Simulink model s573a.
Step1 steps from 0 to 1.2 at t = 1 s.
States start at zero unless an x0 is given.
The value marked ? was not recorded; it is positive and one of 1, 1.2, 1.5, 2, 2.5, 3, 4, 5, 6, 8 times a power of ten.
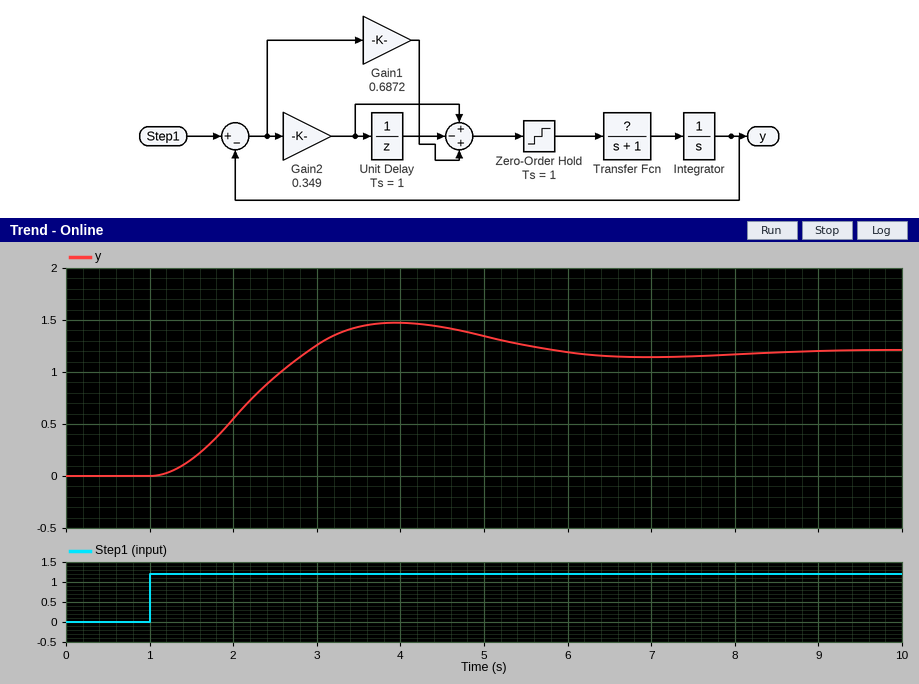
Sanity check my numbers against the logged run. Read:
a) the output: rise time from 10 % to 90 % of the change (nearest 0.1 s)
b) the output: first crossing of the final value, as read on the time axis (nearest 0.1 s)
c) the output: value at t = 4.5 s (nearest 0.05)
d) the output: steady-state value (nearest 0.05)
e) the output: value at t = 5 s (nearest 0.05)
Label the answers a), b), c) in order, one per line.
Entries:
a) 1.3 s
b) 2.9 s
c) 1.45
d) 1.20
e) 1.35
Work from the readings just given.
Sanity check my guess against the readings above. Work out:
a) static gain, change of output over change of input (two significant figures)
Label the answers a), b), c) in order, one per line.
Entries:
a) 1.0
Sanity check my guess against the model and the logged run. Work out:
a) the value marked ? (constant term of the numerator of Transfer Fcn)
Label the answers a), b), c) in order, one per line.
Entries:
a) 1.2
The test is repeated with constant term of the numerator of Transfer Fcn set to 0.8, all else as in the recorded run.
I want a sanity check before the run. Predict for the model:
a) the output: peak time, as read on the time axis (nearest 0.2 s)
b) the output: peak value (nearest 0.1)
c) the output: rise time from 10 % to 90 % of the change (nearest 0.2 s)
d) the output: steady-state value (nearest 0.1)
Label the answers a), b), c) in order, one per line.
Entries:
a) 5.2 s
b) 1.3
c) 2.0 s
d) 1.2
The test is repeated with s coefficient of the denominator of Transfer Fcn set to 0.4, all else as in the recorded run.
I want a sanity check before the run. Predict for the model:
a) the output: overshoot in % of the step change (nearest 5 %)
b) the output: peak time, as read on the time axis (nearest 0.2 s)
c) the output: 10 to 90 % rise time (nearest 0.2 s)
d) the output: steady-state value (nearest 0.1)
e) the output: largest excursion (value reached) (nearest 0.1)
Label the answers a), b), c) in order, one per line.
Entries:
a) 10 %
b) 2.8 s
c) 0.8 s
d) 1.2
e) 1.3
